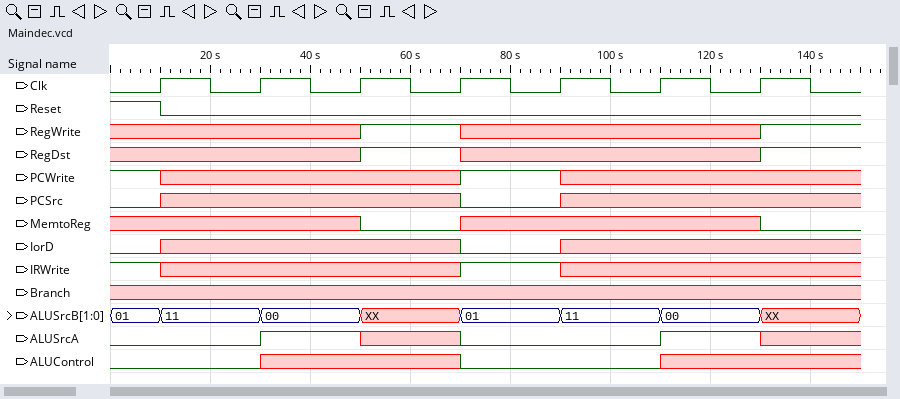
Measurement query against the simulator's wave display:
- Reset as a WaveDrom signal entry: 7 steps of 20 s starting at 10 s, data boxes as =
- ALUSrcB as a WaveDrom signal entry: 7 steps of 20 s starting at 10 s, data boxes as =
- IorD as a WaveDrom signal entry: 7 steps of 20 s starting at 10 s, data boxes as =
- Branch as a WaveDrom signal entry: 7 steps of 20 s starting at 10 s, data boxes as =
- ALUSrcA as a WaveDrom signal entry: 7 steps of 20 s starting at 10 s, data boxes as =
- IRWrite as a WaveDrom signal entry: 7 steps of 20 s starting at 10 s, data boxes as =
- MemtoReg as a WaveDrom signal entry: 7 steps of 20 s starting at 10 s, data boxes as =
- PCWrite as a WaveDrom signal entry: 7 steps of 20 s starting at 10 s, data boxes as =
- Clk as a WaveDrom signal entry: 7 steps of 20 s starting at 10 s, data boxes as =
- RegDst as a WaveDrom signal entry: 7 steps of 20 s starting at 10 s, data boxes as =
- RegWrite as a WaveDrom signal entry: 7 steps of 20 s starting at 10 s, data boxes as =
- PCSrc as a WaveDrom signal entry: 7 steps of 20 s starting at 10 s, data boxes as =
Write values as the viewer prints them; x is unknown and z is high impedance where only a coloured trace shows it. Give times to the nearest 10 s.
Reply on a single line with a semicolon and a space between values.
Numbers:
{name: 'Reset', wave: '0......'}; {name: 'ALUSrcB', wave: '==x===x', data: '11 00 01 11 00'}; {name: 'IorD', wave: 'x..0x..'}; {name: 'Branch', wave: 'x......'}; {name: 'ALUSrcA', wave: '01x0.1x'}; {name: 'IRWrite', wave: 'x..1x..'}; {name: 'MemtoReg', wave: 'x.0x..0'}; {name: 'PCWrite', wave: 'x..1x..'}; {name: 'Clk', wave: 'p......'}; {name: 'RegDst', wave: 'x.1x..1'}; {name: 'RegWrite', wave: 'x.1x..1'}; {name: 'PCSrc', wave: 'x..0x..'}
